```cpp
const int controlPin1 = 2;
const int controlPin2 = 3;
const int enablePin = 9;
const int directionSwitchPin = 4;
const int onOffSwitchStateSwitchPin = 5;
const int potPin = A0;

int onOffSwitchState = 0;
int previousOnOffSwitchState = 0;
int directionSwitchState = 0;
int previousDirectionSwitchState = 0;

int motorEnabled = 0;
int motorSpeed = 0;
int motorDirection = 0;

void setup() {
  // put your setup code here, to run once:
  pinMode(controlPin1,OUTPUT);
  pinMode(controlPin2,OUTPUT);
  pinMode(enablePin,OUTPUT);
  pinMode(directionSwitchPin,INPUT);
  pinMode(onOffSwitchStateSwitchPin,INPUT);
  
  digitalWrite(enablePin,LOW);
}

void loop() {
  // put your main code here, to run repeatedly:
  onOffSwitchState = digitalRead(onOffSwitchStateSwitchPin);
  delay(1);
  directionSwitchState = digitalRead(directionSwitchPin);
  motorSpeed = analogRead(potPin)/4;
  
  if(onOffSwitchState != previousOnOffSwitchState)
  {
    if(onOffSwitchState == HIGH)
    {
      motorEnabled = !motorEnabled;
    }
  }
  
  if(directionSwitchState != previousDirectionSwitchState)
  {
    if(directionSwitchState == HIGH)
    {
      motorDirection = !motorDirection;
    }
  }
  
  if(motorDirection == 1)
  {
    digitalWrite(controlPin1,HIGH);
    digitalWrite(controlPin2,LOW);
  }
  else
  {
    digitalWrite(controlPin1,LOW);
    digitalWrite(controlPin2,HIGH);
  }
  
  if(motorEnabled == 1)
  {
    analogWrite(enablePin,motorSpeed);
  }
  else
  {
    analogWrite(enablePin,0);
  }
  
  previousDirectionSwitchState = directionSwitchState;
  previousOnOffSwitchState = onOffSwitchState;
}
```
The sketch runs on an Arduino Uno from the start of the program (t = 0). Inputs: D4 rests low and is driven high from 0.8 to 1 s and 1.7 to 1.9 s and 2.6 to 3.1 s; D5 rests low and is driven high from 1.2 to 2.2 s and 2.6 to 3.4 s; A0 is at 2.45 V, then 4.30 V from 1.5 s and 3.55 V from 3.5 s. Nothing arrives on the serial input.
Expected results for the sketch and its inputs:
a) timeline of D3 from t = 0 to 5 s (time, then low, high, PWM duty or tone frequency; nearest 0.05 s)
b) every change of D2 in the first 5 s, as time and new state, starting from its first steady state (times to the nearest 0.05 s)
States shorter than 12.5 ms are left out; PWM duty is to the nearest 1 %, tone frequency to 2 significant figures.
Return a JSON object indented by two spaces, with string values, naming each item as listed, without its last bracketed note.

{
  "timeline of D3 from t = 0 to 5 s": "0 s high; 0.8 s low; 1.7 s high; 2.6 s low",
  "every change of D2 in the first 5 s, as time and new state, starting from its first steady state": "0 s low; 0.8 s high; 1.7 s low; 2.6 s high"
}
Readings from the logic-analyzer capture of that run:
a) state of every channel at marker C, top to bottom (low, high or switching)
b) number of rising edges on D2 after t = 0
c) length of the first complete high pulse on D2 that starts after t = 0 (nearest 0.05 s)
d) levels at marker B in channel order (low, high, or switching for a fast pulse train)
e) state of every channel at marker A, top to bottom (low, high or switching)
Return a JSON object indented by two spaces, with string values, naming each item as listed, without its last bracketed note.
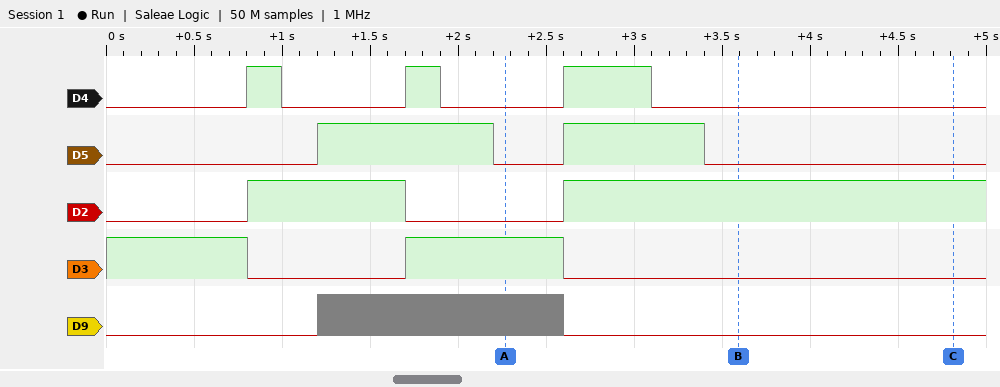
{
  "state of every channel at marker C, top to bottom": "D4 low, D5 low, D2 high, D3 low, D9 low",
  "number of rising edges on D2 after t = 0": "2",
  "length of the first complete high pulse on D2 that starts after t = 0": "0.90 s",
  "levels at marker B in channel order": "D4 low, D5 low, D2 high, D3 low, D9 low",
  "state of every channel at marker A, top to bottom": "D4 low, D5 low, D2 low, D3 high, D9 switching"
}
